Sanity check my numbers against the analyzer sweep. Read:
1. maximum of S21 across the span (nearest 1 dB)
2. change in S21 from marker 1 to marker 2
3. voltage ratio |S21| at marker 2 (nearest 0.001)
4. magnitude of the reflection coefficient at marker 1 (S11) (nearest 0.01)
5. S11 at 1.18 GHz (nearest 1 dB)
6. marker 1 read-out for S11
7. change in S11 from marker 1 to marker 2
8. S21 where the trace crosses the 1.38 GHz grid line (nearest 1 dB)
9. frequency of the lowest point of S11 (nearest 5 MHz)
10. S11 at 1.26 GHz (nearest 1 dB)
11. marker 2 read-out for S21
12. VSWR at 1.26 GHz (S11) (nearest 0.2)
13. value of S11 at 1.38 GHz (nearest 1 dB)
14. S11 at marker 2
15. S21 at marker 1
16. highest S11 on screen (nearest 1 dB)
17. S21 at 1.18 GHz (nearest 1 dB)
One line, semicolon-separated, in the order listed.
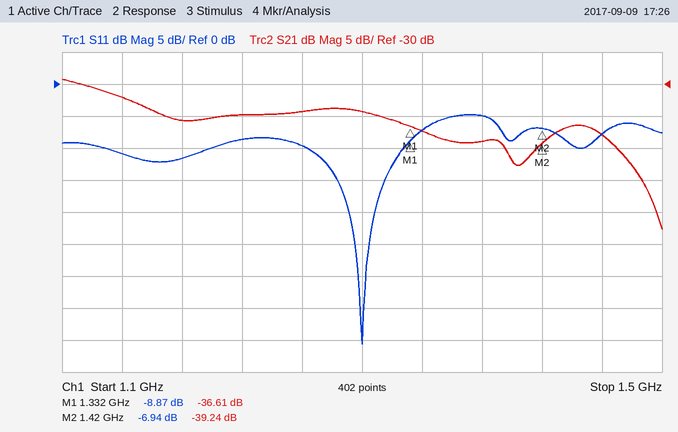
-29 dB; -2.63 dB; 0.011; 0.36; -12 dB; -8.87 dB; 1.93 dB; -39 dB; 1.300 GHz; -10 dB; -39.24 dB; 2.0; -5 dB; -6.94 dB; -36.61 dB; -5 dB; -36 dB
